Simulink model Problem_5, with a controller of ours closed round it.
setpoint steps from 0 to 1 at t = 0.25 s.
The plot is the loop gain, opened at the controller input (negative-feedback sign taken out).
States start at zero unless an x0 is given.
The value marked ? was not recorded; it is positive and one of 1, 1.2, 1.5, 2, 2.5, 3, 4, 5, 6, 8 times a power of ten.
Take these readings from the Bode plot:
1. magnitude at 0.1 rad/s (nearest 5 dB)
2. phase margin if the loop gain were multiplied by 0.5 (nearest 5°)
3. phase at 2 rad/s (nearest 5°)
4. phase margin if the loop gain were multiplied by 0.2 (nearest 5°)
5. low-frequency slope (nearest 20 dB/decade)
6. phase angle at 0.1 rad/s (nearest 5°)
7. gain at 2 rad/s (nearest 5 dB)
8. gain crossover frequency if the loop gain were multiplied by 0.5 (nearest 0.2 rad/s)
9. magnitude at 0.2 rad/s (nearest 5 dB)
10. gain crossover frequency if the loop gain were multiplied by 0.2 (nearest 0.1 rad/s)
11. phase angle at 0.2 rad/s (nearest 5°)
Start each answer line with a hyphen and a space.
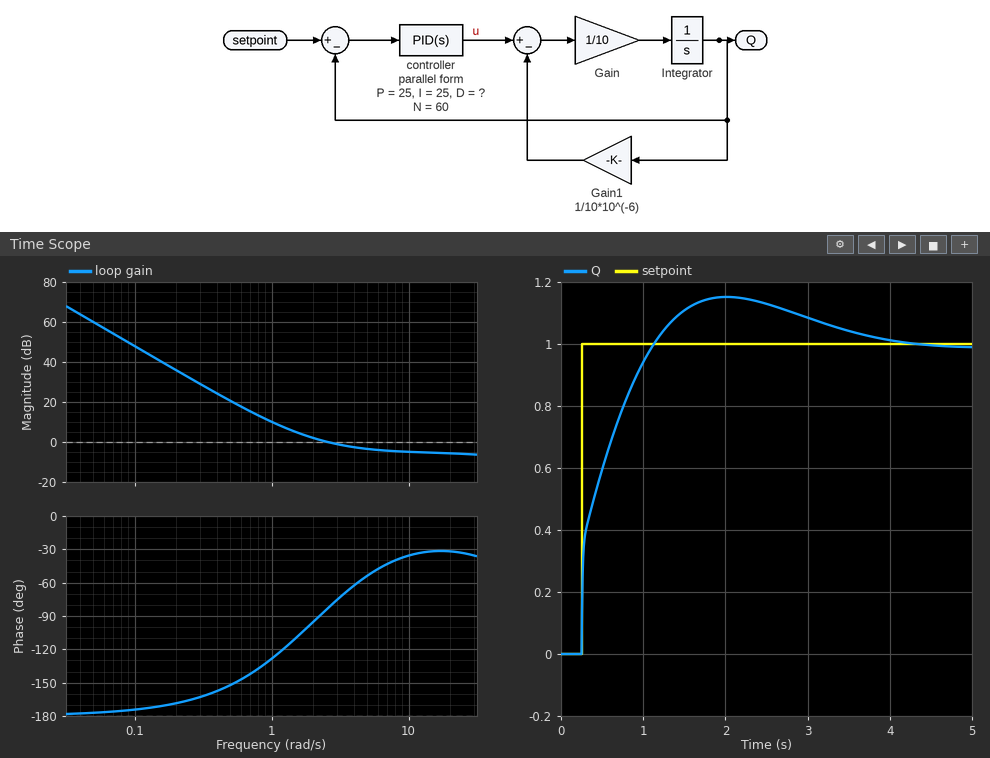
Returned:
- 50 dB
- 65°
- -95°
- 40°
- -40 dB/decade
- -175°
- 0 dB
- 1.4 rad/s
- 35 dB
- 0.8 rad/s
- -170°
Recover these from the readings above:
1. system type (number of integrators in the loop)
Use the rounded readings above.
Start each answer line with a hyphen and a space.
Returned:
- 2
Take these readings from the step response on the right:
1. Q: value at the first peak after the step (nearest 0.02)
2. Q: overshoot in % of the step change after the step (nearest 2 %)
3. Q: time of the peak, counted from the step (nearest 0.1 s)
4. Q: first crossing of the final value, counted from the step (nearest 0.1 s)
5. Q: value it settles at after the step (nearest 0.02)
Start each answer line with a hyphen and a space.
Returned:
- 1.16
- 16 %
- 1.8 s
- 0.9 s
- 1.00
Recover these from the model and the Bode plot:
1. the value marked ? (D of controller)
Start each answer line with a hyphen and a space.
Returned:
- 5
